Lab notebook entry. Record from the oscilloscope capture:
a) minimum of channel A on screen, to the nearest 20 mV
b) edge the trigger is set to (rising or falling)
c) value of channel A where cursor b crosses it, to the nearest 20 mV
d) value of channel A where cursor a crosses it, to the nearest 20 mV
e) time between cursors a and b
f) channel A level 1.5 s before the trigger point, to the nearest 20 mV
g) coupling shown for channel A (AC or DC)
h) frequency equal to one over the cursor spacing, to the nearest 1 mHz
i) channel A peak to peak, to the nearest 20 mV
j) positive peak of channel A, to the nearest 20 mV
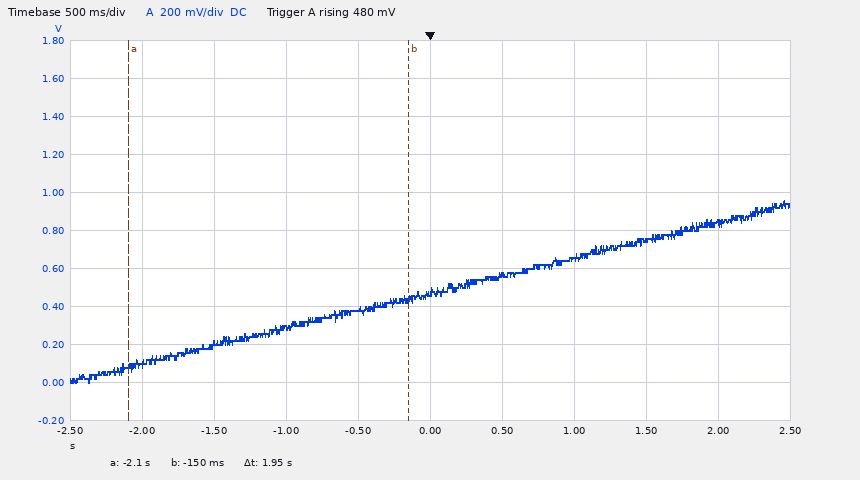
0 mV
rising
440 mV
80 mV
1.95 s
200 mV
DC
513 mHz
960 mV
960 mV
